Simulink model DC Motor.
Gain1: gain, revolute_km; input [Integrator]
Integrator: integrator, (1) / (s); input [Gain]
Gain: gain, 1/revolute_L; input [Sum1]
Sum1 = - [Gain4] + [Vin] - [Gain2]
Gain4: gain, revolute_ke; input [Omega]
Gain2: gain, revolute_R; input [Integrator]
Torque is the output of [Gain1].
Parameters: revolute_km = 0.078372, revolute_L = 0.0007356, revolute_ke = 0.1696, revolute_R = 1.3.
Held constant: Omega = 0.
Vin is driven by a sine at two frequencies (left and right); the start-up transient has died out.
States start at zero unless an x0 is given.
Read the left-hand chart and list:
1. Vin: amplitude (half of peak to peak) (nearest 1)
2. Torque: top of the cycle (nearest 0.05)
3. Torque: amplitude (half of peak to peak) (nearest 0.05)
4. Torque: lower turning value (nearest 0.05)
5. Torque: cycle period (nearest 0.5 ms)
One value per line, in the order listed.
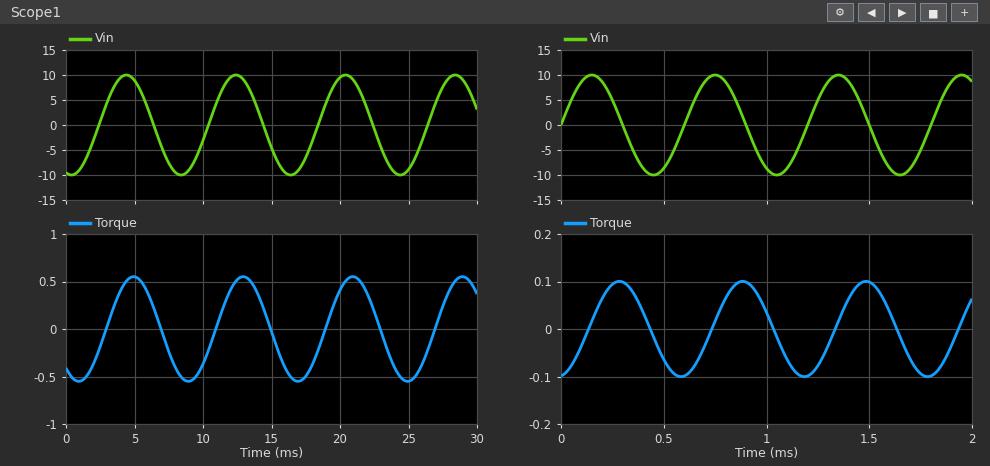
10
0.55
0.55
-0.55
8.0 ms
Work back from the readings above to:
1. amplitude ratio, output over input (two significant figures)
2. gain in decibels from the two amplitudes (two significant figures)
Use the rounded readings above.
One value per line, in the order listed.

0.055
-25 dB
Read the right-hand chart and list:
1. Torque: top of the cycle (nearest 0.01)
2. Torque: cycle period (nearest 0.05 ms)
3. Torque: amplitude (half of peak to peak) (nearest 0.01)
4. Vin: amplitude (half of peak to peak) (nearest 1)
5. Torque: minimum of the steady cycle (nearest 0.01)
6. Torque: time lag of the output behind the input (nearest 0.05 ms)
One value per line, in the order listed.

0.10
0.60 ms
0.10
10
-0.10
0.15 ms
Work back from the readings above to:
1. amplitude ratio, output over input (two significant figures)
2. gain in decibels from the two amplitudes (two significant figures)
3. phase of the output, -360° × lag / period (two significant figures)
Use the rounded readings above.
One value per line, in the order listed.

0.010
-40 dB
-90°
